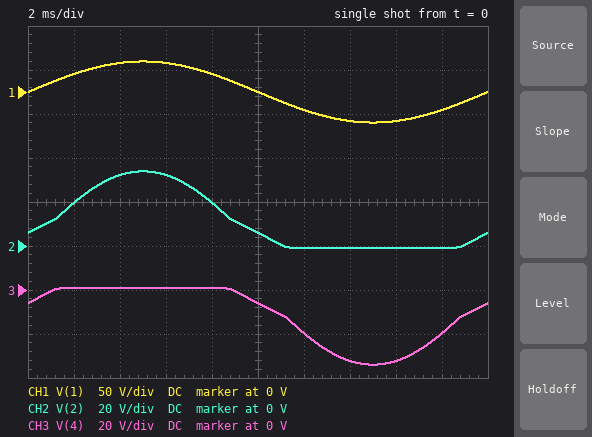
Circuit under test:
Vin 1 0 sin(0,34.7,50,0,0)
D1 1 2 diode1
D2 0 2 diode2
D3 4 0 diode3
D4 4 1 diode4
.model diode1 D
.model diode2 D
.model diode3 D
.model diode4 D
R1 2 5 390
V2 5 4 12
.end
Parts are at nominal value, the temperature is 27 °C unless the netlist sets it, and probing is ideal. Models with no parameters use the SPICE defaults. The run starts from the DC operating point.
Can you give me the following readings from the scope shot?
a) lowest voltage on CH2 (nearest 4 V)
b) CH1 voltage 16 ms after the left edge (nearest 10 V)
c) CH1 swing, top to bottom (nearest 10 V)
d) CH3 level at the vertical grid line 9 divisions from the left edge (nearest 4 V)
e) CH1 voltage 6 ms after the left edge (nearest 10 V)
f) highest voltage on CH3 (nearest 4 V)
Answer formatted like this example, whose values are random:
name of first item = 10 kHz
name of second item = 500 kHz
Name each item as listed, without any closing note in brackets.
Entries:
lowest voltage on CH2 = 0 V
CH1 voltage 16 ms after the left edge = -30 V
CH1 swing, top to bottom = 70 V
CH3 level at the vertical grid line 9 divisions from the left edge = -20 V
CH1 voltage 6 ms after the left edge = 30 V
highest voltage on CH3 = 0 V
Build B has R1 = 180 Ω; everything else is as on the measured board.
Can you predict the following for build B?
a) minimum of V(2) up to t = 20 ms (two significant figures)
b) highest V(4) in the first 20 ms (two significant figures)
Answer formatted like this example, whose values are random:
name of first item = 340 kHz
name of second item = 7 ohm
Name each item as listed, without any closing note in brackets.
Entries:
minimum of V(2) up to t = 20 ms = -780 mV
highest V(4) in the first 20 ms = 780 mV
